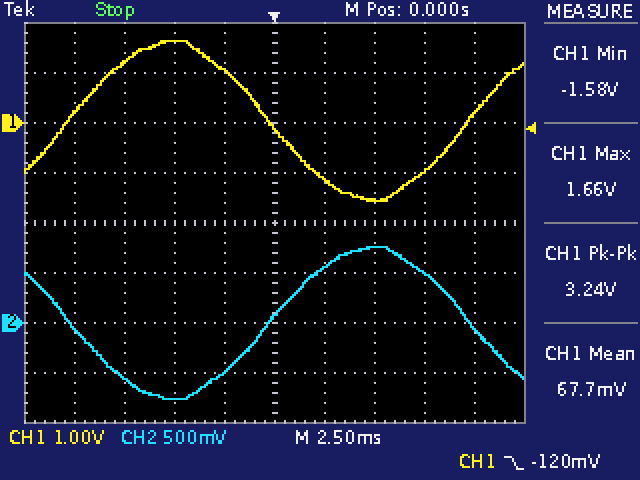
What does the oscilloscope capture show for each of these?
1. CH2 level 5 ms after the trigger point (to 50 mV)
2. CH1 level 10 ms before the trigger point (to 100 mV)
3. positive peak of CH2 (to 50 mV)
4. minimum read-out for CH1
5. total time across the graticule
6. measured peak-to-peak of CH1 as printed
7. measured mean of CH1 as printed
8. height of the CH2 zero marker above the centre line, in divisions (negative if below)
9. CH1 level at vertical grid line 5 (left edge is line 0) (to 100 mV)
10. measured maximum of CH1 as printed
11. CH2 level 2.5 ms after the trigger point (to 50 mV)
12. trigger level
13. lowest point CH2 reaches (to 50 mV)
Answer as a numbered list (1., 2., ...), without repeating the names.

1. 750 mV
2. 200 mV
3. 750 mV
4. -1.58 V
5. 25 ms
6. 3.24 V
7. 67.7 mV
8. -2.0 div
9. -100 mV
10. 1.66 V
11. 550 mV
12. -120 mV
13. -750 mV
